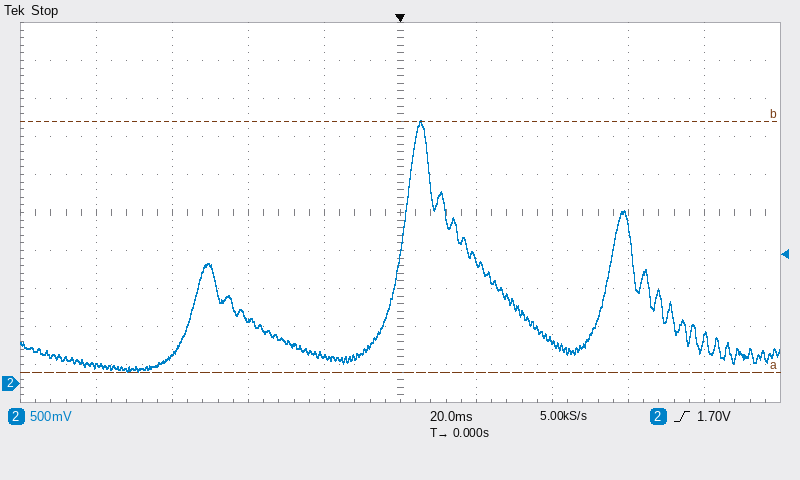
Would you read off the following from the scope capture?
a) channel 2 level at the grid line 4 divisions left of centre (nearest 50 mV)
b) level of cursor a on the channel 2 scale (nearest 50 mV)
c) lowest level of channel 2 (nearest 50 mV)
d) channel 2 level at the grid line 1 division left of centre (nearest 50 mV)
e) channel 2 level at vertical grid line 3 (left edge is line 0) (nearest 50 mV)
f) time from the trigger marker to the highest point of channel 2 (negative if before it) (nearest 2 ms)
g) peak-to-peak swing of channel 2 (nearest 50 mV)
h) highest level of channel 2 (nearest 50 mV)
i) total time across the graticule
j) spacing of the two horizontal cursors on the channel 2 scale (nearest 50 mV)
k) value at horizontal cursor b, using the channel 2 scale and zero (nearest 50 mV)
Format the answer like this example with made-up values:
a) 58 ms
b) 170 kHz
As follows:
a) 250 mV
b) 150 mV
c) 150 mV
d) 350 mV
e) 850 mV
f) +6 ms
g) 3.30 V
h) 3.45 V
i) 200 ms
j) 3.30 V
k) 3.45 V
